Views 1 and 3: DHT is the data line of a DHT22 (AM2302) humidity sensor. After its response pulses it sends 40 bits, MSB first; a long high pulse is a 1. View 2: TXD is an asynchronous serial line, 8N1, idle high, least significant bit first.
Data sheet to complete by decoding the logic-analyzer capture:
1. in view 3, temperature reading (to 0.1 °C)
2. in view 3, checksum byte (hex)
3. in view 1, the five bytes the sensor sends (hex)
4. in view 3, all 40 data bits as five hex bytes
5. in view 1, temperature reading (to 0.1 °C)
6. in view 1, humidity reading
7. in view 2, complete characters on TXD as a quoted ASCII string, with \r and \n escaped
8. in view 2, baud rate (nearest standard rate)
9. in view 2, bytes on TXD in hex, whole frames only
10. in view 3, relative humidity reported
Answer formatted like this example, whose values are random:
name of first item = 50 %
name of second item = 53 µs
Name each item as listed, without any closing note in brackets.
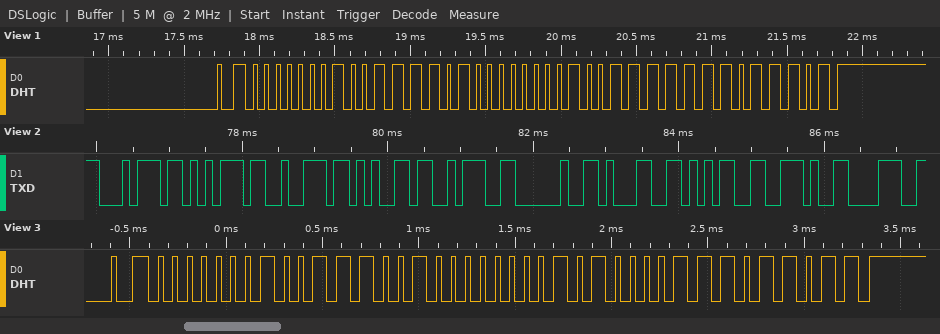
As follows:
in view 3, temperature reading = 16.1 °C
in view 3, checksum byte = 0xDB
in view 1, the five bytes the sensor sends = 01 3D 00 9F DD
in view 3, all 40 data bits as five hex bytes = 01 39 00 A1 DB
in view 1, temperature reading = 15.9 °C
in view 1, humidity reading = 31.7 %
in view 2, complete characters on TXD as a quoted ASCII string, with \r and \n escaped = "ture: 15.8"
in view 2, baud rate = 9600 baud
in view 2, bytes on TXD in hex, whole frames only = 74 75 72 65 3A 20 31 35 2E 38
in view 3, relative humidity reported = 31.3 %
